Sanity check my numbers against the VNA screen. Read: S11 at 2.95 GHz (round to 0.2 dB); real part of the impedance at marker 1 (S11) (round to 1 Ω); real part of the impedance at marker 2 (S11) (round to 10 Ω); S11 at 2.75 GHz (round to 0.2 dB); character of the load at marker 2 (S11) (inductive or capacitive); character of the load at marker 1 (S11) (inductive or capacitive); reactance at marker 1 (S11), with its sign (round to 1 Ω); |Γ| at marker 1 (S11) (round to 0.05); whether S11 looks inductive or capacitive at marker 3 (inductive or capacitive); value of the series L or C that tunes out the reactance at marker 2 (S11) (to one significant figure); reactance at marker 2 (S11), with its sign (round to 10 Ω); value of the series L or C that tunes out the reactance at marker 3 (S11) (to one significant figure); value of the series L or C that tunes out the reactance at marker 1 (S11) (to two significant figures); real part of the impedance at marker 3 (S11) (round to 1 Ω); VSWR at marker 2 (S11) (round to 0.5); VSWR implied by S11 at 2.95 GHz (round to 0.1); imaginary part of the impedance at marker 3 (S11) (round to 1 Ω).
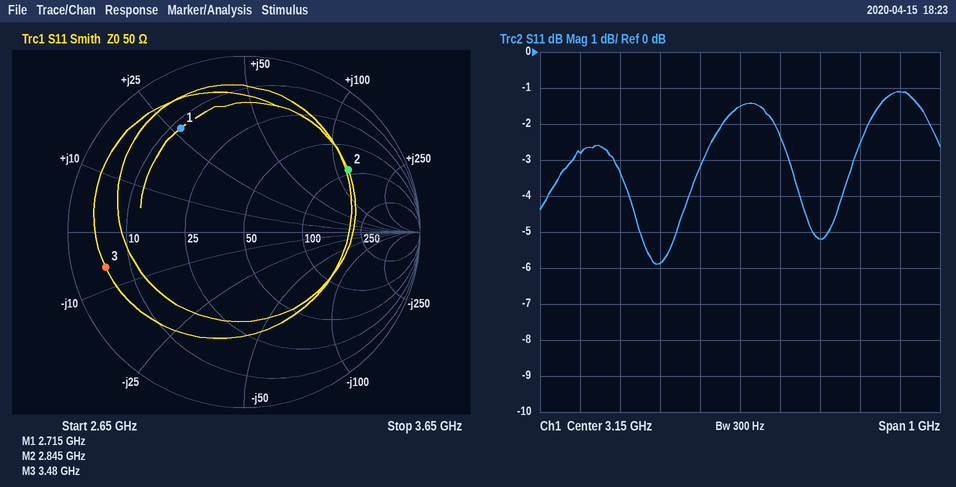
-5.8 dB
12 Ω
90 Ω
-2.8 dB
inductive
inductive
+27 Ω
0.70
capacitive
500 fF
+120 Ω
300 pH
2.2 pF
5 Ω
5.5
3.1
-6 Ω
